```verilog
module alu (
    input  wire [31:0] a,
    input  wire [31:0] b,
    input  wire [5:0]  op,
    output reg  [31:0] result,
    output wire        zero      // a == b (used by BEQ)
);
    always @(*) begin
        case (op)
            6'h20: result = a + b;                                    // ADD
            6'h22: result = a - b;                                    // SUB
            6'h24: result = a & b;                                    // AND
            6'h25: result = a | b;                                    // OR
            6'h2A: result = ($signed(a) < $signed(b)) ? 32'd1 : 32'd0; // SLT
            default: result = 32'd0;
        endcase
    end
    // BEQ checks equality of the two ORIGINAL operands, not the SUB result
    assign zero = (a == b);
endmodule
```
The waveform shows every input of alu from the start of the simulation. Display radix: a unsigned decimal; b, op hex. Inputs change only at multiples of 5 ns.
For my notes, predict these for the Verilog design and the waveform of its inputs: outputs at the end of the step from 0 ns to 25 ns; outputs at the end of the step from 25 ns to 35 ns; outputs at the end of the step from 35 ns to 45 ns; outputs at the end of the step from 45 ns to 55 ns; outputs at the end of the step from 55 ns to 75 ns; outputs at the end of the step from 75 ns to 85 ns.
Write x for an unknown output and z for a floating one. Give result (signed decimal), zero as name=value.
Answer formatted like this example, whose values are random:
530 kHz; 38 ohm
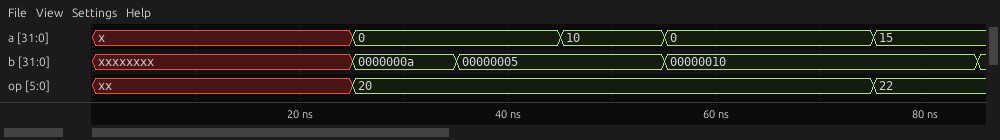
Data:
result=x, zero=x; result=10, zero=0; result=5, zero=0; result=15, zero=0; result=16, zero=0; result=-1, zero=0
